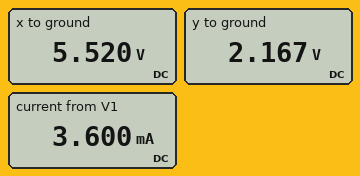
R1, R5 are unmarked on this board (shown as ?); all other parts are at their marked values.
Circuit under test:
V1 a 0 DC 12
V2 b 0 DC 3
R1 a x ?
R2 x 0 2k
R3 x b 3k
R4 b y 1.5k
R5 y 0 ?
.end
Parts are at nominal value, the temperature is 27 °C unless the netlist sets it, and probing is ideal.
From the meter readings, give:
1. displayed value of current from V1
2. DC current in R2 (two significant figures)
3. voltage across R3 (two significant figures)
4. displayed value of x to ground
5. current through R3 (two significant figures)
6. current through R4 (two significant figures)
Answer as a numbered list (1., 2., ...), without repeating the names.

1. 3.600 mA
2. 2.8 mA
3. 2.5 V
4. 5.520 V
5. 840 µA
6. 560 µA
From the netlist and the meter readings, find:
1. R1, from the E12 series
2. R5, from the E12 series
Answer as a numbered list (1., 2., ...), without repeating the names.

1. 1.8 kΩ
2. 3.9 kΩ
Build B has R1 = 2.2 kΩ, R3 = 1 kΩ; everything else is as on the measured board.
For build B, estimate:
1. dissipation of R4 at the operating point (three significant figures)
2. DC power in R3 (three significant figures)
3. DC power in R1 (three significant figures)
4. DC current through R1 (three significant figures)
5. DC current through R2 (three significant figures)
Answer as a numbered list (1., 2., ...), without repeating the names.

1. 463 µW
2. 1.76 mW
3. 26.8 mW
4. 3.49 mA
5. 2.16 mA
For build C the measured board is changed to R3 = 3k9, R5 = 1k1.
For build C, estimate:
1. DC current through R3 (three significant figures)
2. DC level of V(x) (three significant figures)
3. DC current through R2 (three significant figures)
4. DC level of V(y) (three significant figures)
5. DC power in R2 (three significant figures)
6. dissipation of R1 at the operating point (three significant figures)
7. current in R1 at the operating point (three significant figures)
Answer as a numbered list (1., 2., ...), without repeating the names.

1. 684 µA
2. 5.67 V
3. 2.83 mA
4. 1.27 V
5. 16.1 mW
6. 22.3 mW
7. 3.52 mA
